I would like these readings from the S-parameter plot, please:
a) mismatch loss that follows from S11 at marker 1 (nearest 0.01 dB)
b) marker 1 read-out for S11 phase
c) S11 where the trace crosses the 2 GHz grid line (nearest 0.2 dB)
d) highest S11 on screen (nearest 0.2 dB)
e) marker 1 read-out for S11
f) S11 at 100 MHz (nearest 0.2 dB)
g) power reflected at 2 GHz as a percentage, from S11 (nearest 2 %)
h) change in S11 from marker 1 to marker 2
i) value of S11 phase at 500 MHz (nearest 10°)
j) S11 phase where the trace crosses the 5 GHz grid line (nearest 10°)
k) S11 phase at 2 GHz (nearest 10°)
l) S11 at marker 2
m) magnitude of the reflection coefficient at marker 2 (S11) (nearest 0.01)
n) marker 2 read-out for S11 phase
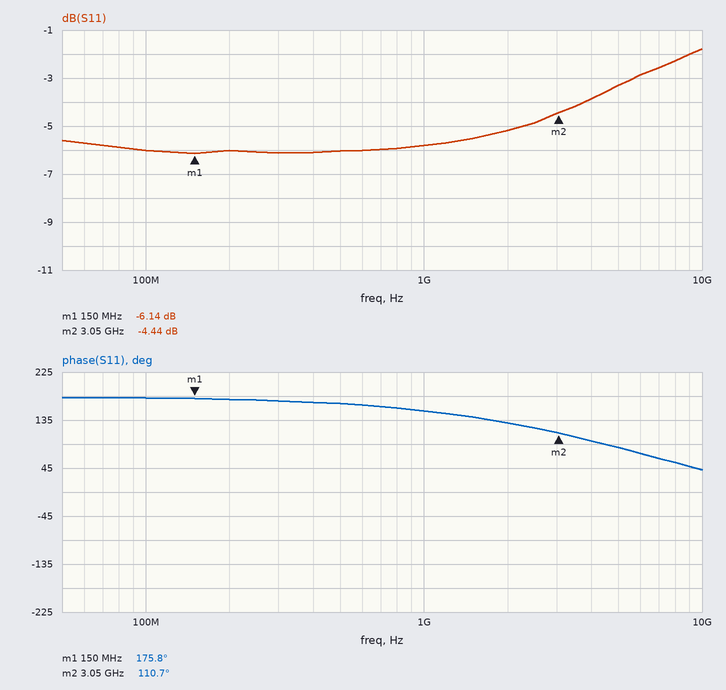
1.21 dB
175.8°
-5.2 dB
-1.8 dB
-6.14 dB
-6.0 dB
30 %
1.70 dB
170°
80°
130°
-4.44 dB
0.60
110.7°
